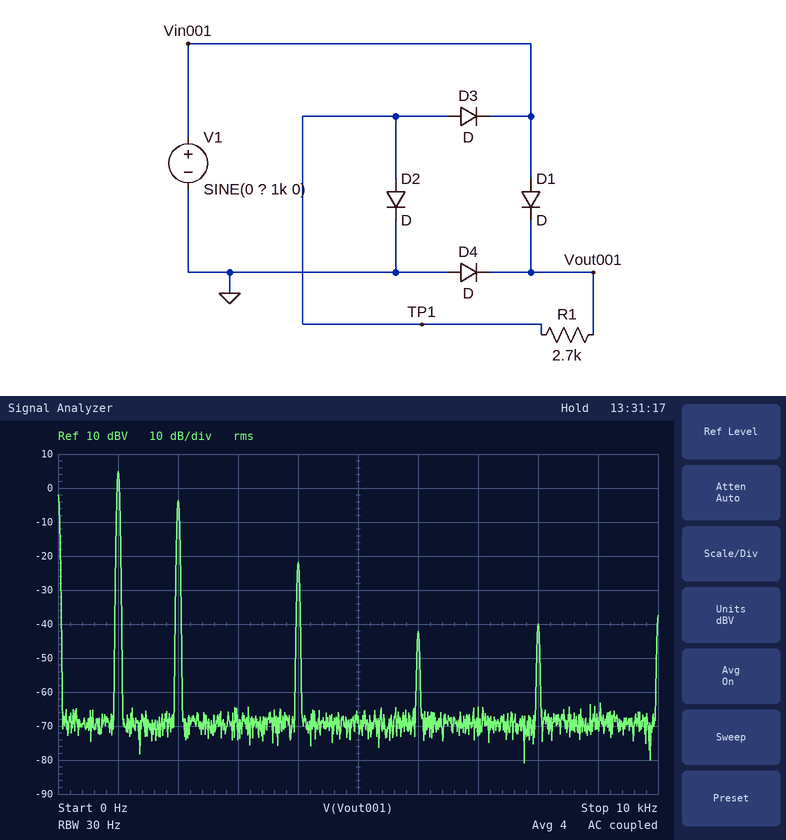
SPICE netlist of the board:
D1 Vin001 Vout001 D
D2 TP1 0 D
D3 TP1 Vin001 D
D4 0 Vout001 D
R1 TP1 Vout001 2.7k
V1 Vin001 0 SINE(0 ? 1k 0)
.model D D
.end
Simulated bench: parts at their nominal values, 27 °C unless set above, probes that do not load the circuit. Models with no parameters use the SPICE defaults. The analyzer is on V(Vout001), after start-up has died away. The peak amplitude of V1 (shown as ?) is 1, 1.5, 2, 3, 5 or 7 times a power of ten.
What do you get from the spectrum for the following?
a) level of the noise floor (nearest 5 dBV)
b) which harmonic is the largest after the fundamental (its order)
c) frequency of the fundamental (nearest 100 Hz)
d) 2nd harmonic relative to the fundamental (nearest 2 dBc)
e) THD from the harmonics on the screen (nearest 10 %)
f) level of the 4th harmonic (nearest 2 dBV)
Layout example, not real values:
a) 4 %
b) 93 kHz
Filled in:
a) -70 dBV
b) 2
c) 1.0 kHz
d) -8 dBc
e) 40 %
f) -22 dBV
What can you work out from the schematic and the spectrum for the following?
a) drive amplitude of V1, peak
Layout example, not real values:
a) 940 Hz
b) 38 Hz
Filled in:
a) 5 V
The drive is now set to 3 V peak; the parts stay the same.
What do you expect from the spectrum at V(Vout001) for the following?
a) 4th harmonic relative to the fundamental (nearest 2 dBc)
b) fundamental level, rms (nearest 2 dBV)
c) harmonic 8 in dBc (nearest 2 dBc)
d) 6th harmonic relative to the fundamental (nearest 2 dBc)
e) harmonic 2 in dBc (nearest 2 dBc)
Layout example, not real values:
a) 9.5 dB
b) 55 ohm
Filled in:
a) -54 dBc
b) 0 dBV
c) -36 dBc
d) -34 dBc
e) -10 dBc
